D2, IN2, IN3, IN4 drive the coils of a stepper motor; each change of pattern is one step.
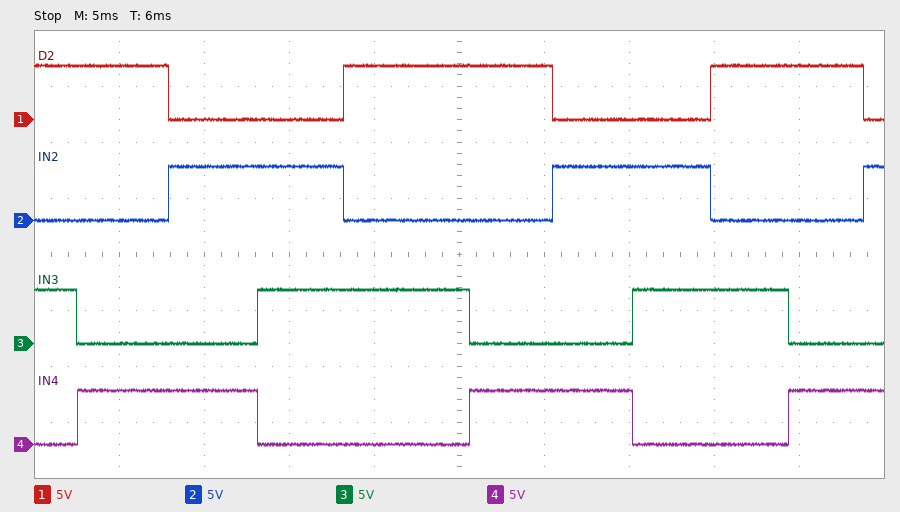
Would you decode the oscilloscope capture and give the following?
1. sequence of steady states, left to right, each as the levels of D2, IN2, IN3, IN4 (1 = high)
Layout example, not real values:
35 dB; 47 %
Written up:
1010 1001 0101 0110 1010 1001 0101 0110 1010 1001 0101
